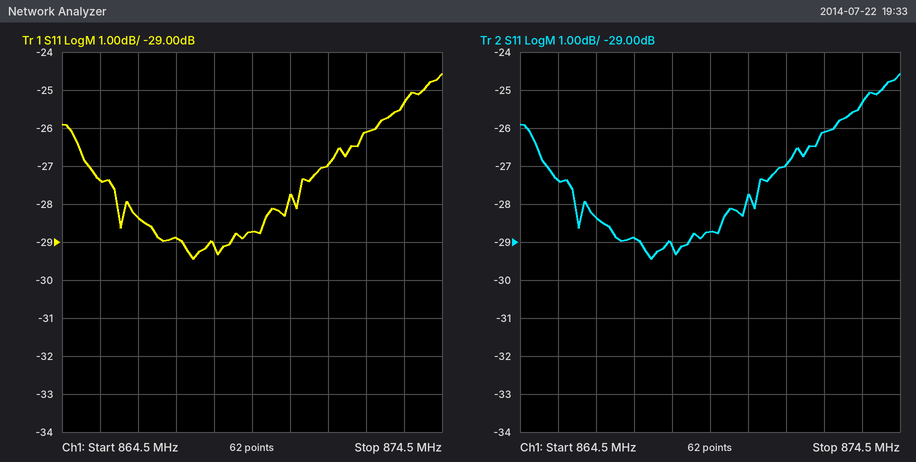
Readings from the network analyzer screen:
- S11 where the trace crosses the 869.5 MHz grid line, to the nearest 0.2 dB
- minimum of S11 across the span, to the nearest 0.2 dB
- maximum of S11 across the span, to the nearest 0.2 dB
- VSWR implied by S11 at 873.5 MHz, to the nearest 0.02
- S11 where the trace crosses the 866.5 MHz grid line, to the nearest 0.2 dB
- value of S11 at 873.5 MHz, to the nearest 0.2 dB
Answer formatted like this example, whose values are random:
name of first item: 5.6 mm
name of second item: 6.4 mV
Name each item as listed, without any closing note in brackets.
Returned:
S11 where the trace crosses the 869.5 MHz grid line, to the nearest 0.2 dB: -28.8 dB
minimum of S11 across the span, to the nearest 0.2 dB: -29.4 dB
maximum of S11 across the span, to the nearest 0.2 dB: -24.6 dB
VSWR implied by S11 at 873.5 MHz, to the nearest 0.02: 1.12
S11 where the trace crosses the 866.5 MHz grid line, to the nearest 0.2 dB: -28.4 dB
value of S11 at 873.5 MHz, to the nearest 0.2 dB: -25.4 dB
